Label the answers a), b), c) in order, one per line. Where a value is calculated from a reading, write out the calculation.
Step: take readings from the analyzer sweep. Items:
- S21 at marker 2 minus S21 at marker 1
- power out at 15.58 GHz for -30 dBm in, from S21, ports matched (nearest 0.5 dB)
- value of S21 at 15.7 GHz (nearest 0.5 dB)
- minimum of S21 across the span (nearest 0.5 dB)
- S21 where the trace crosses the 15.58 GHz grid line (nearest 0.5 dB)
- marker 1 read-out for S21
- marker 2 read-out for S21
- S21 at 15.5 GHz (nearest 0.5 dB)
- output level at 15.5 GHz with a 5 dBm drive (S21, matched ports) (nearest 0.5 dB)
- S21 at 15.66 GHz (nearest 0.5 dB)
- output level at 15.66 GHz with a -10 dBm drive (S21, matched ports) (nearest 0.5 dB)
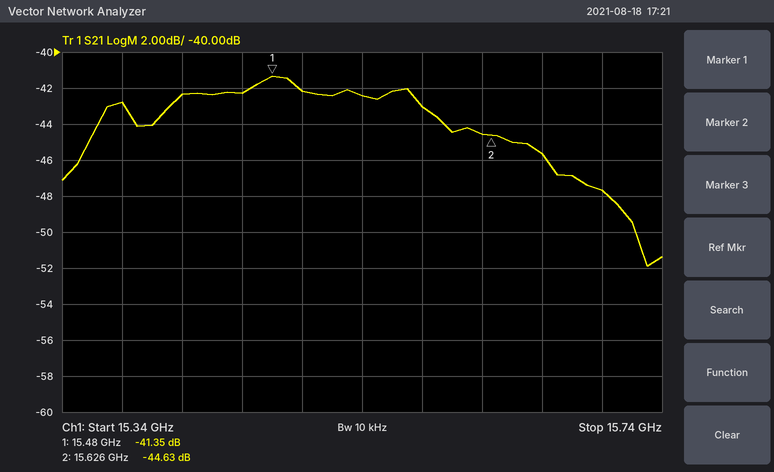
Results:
a) -44.63 − (-41.35) = -3.28 dB
b) -30 dBm + (-43.0 dB) = -73.0 dBm
c) -47.5 dB
d) -52.0 dB
e) -43.0 dB
f) -41.35 dB
g) -44.63 dB
h) -42.0 dB
i) 5 dBm + (-42.0 dB) = -37.0 dBm
j) -45.5 dB
k) -10 dBm + (-45.5 dB) = -55.5 dBm
